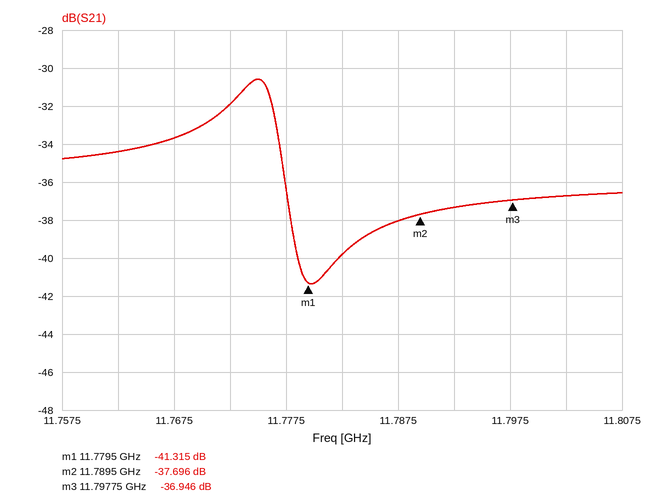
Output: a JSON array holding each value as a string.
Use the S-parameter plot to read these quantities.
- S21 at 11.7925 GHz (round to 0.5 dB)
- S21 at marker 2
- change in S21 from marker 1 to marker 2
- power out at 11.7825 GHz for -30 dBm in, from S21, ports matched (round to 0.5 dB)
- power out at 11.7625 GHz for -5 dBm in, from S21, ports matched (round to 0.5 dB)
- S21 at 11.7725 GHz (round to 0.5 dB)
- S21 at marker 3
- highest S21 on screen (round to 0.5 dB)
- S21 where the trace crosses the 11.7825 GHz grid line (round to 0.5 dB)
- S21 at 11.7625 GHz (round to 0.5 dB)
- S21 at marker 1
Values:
["-37.5 dB", "-37.696 dB", "3.619 dB", "-70.0 dBm", "-39.5 dBm", "-32.0 dB", "-36.946 dB", "-30.5 dB", "-40.0 dB", "-34.5 dB", "-41.315 dB"]
